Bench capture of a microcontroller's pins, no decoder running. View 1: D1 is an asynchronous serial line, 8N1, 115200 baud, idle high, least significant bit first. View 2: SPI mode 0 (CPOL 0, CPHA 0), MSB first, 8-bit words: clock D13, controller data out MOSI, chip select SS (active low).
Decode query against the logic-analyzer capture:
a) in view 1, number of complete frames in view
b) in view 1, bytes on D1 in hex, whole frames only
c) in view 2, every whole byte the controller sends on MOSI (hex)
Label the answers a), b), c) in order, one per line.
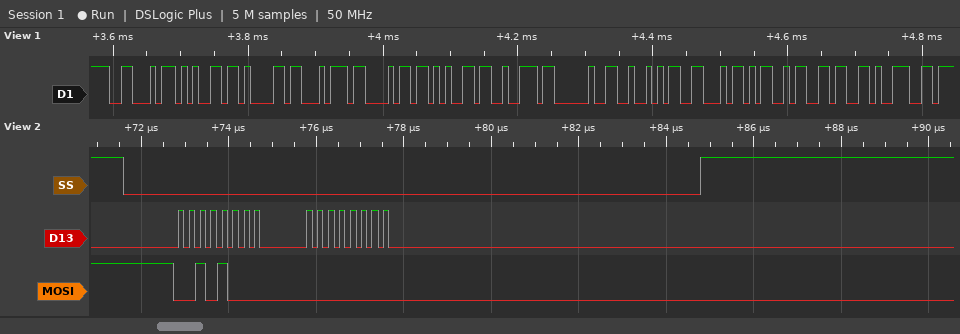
a) 13
b) 46 65 61 74 68 65 72 20 52 46 4D 36 39
c) 28 00
